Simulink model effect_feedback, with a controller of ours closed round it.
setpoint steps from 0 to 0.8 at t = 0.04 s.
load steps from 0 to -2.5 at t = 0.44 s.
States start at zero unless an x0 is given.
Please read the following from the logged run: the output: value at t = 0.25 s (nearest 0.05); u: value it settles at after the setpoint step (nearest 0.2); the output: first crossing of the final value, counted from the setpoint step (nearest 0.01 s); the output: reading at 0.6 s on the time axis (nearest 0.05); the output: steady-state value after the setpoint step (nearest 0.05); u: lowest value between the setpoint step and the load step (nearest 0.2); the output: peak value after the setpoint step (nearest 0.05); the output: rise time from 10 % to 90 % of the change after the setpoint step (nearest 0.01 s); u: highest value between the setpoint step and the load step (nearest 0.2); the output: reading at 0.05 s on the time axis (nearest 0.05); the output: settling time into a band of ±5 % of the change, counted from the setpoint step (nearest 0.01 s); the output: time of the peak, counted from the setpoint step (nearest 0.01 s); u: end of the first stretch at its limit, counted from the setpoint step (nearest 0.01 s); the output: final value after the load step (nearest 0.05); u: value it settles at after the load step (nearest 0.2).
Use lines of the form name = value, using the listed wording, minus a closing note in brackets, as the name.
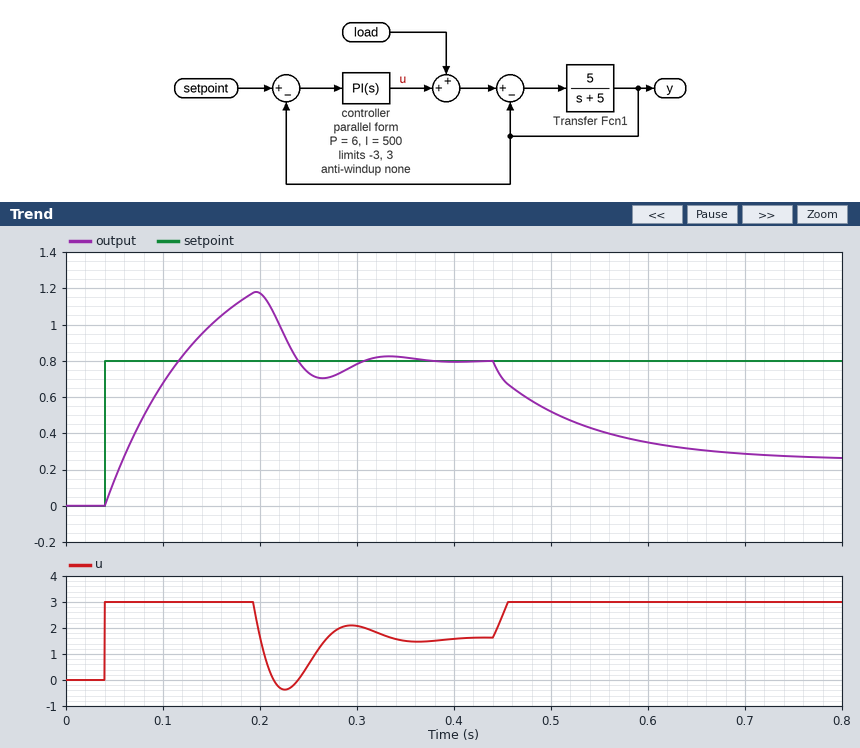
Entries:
the output: value at t = 0.25 s = 0.75
u: value it settles at after the setpoint step = 1.6
the output: first crossing of the final value, counted from the setpoint step = 0.08 s
the output: reading at 0.6 s on the time axis = 0.35
the output: steady-state value after the setpoint step = 0.80
u: lowest value between the setpoint step and the load step = -0.4
the output: peak value after the setpoint step = 1.20
the output: rise time from 10 % to 90 % of the change after the setpoint step = 0.06 s
u: highest value between the setpoint step and the load step = 3.0
the output: reading at 0.05 s on the time axis = 0.15
the output: settling time into a band of ±5 % of the change, counted from the setpoint step = 0.25 s
the output: time of the peak, counted from the setpoint step = 0.16 s
u: end of the first stretch at its limit, counted from the setpoint step = 0.15 s
the output: final value after the load step = 0.25
u: value it settles at after the load step = 3.0
